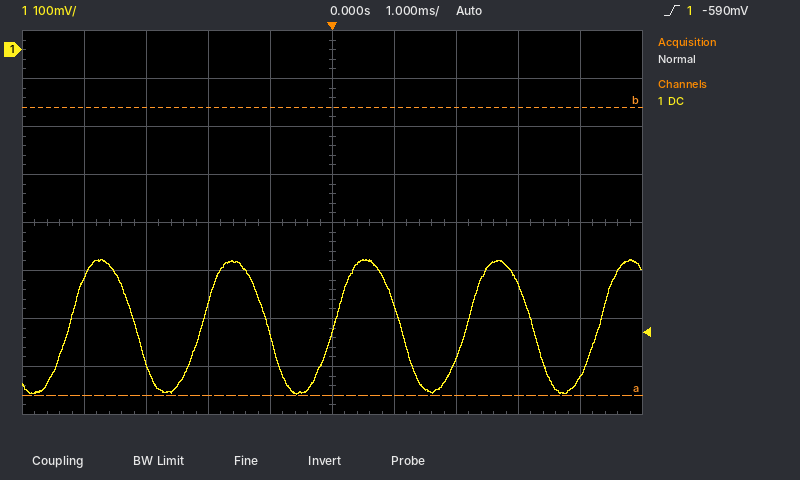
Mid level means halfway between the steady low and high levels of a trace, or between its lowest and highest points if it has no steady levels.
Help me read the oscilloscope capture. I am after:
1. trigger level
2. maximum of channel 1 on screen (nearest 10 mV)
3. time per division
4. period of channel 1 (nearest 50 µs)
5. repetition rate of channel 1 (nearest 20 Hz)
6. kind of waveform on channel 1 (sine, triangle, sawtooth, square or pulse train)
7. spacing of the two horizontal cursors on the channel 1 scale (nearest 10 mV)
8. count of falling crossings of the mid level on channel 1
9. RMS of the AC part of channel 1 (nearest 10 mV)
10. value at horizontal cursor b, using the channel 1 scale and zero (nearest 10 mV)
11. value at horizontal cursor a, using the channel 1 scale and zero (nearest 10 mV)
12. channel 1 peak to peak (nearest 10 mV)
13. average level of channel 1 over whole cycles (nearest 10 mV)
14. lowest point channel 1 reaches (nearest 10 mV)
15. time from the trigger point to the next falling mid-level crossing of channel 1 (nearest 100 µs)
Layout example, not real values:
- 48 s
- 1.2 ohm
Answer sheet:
- -590 mV
- -440 mV
- 1 ms
- 2.15 ms
- 460 Hz
- sine
- 600 mV
- 4
- 100 mV
- -120 mV
- -720 mV
- 280 mV
- -580 mV
- -720 mV
- 1.1 ms
